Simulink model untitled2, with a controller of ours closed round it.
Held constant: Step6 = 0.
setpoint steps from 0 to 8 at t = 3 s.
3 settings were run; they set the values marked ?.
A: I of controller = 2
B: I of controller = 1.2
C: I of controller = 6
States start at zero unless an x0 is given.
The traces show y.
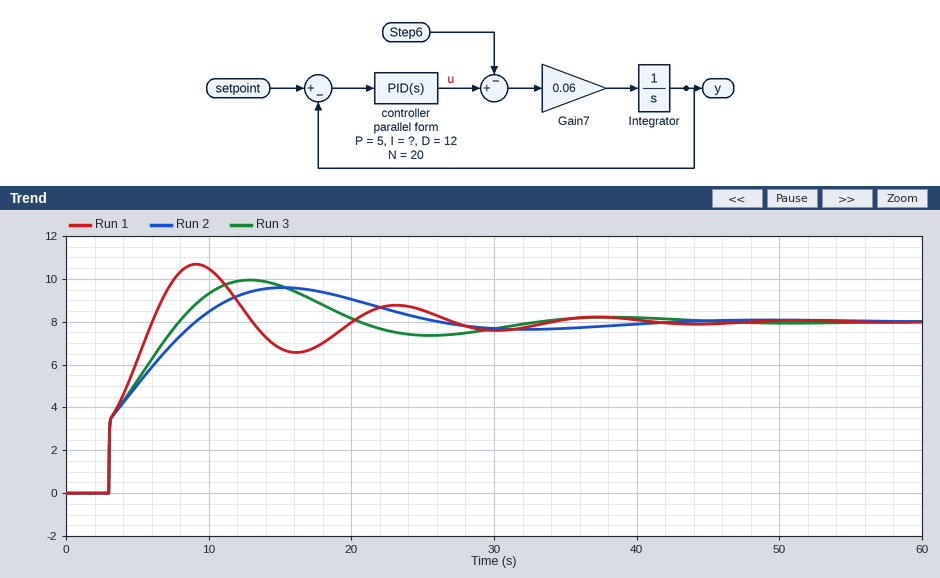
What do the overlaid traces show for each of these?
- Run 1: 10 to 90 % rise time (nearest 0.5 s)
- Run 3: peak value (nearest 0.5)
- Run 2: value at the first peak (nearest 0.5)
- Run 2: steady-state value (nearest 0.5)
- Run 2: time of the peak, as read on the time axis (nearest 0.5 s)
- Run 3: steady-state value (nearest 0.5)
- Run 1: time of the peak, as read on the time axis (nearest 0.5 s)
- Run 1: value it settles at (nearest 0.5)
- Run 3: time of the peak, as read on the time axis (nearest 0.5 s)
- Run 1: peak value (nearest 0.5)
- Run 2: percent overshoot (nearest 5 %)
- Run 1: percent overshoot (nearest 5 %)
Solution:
2.5 s
10.0
9.5
8.0
15.0 s
8.0
9.0 s
8.0
13.0 s
10.5
20 %
35 %
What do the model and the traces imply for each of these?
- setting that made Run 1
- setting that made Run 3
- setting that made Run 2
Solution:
C
A
B
